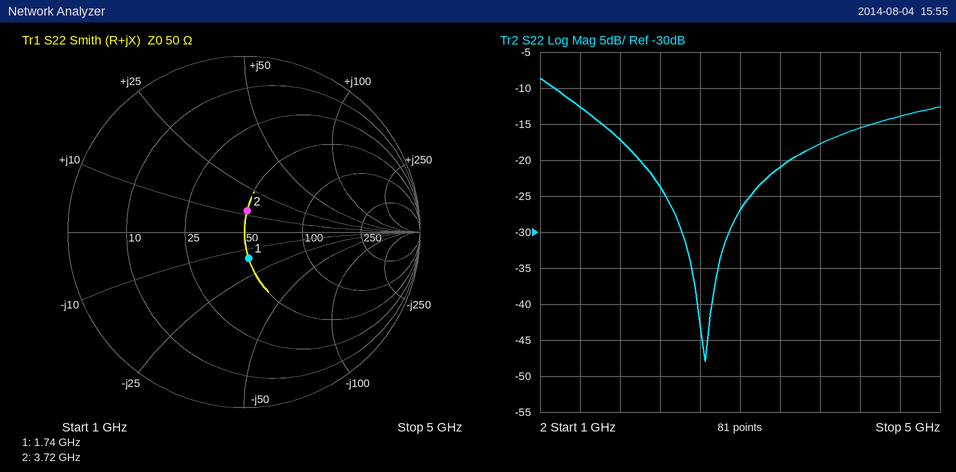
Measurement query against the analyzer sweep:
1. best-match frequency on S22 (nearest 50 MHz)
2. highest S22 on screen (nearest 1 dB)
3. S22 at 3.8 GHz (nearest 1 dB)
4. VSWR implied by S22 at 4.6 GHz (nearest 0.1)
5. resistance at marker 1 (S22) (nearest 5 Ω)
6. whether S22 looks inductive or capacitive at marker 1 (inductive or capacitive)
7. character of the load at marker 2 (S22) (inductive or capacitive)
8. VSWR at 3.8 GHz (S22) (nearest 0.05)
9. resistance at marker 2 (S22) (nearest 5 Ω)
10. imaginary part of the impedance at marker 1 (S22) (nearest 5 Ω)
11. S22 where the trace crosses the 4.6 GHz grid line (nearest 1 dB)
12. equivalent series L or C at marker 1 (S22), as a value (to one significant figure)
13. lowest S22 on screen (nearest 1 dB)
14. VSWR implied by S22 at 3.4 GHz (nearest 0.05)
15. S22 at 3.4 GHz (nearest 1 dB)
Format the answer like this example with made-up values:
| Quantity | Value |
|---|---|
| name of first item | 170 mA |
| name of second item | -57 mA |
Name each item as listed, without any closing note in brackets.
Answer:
| Quantity | Value |
|---|---|
| best-match frequency on S22 | 2.65 GHz |
| highest S22 on screen | -9 dB |
| S22 at 3.8 GHz | -18 dB |
| VSWR implied by S22 at 4.6 GHz | 1.5 |
| resistance at marker 1 (S22) | 50 Ω |
| whether S22 looks inductive or capacitive at marker 1 | capacitive |
| character of the load at marker 2 (S22) | inductive |
| VSWR at 3.8 GHz (S22) | 1.30 |
| resistance at marker 2 (S22) | 50 Ω |
| imaginary part of the impedance at marker 1 (S22) | -15 Ω |
| S22 where the trace crosses the 4.6 GHz grid line | -14 dB |
| equivalent series L or C at marker 1 (S22), as a value | 6 pF |
| lowest S22 on screen | -48 dB |
| VSWR implied by S22 at 3.4 GHz | 1.20 |
| S22 at 3.4 GHz | -21 dB |
